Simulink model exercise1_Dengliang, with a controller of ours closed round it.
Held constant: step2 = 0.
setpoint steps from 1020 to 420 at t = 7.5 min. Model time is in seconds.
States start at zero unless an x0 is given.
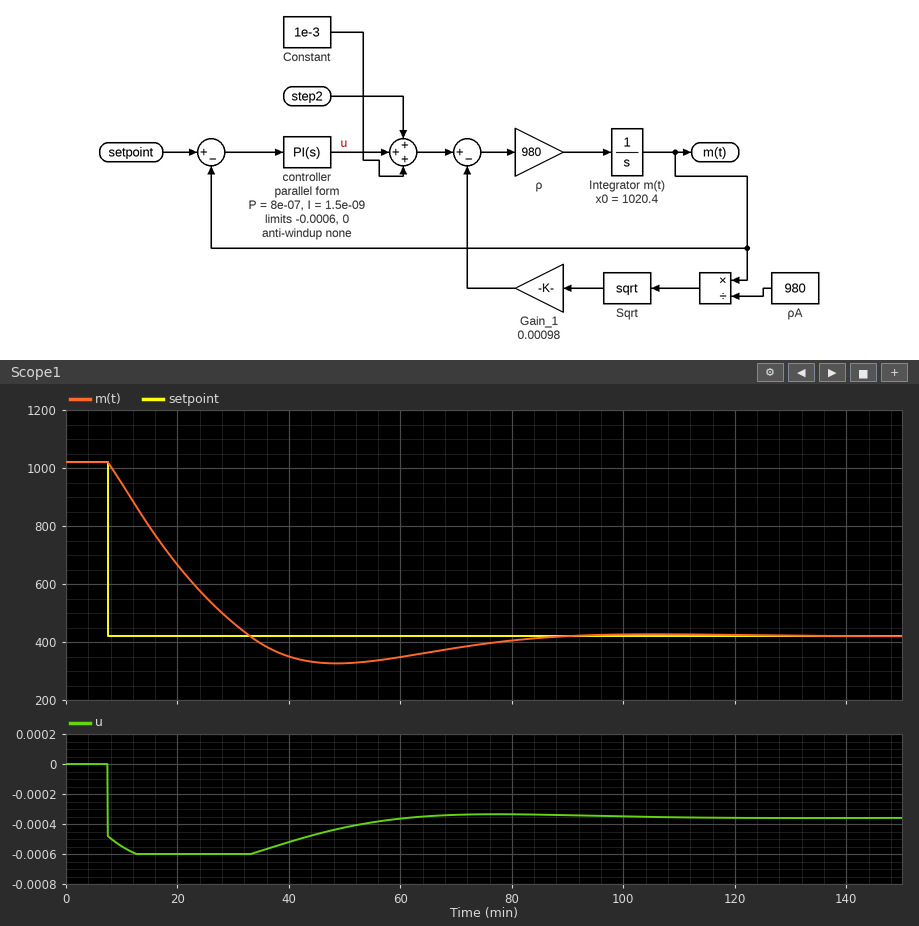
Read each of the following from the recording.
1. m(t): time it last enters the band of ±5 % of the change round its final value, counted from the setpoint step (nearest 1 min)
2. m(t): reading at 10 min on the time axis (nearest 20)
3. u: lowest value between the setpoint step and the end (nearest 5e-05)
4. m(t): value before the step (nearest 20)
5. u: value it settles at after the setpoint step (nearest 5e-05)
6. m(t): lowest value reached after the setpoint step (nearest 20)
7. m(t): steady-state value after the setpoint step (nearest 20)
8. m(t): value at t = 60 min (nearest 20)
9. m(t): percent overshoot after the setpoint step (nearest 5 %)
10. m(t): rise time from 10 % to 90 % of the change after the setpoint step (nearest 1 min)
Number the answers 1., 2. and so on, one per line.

1. 66 min
2. 940
3. -0.00060
4. 1020
5. -0.00035
6. 320
7. 420
8. 340
9. 15 %
10. 20 min
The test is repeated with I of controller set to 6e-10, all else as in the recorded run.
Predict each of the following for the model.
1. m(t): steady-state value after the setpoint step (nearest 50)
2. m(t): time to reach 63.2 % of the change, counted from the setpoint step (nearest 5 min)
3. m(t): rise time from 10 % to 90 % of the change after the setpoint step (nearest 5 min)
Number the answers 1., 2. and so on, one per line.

1. 400
2. 20 min
3. 35 min
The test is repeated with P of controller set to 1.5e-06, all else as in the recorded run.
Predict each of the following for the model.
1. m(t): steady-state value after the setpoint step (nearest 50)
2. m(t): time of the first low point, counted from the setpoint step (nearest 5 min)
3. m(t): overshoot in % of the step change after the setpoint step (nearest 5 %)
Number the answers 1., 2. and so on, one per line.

1. 400
2. 40 min
3. 10 %
